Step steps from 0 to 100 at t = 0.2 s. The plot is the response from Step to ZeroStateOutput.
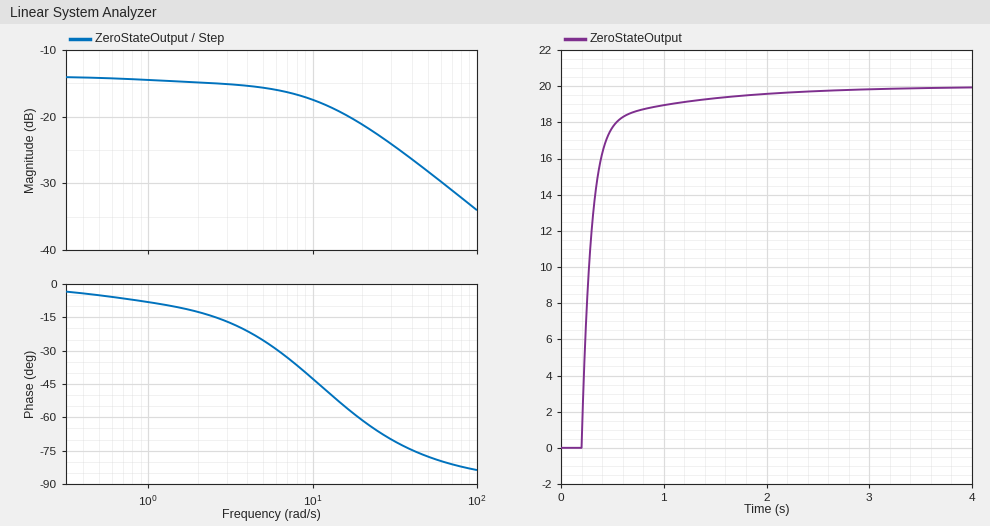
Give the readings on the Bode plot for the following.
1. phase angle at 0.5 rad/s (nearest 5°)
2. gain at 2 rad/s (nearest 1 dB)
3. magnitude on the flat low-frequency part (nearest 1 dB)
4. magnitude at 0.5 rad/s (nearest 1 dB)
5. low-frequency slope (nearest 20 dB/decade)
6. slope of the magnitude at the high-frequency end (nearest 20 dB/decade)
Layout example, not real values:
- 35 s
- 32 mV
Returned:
- -5°
- -15 dB
- -14 dB
- -14 dB
- 0 dB/decade
- -20 dB/decade
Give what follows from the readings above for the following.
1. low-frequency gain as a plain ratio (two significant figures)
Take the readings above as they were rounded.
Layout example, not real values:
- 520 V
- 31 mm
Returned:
- 0.20
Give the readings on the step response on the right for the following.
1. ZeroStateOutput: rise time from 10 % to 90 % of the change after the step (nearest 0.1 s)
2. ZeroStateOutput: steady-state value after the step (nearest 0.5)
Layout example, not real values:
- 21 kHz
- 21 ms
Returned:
- 0.3 s
- 20.0
